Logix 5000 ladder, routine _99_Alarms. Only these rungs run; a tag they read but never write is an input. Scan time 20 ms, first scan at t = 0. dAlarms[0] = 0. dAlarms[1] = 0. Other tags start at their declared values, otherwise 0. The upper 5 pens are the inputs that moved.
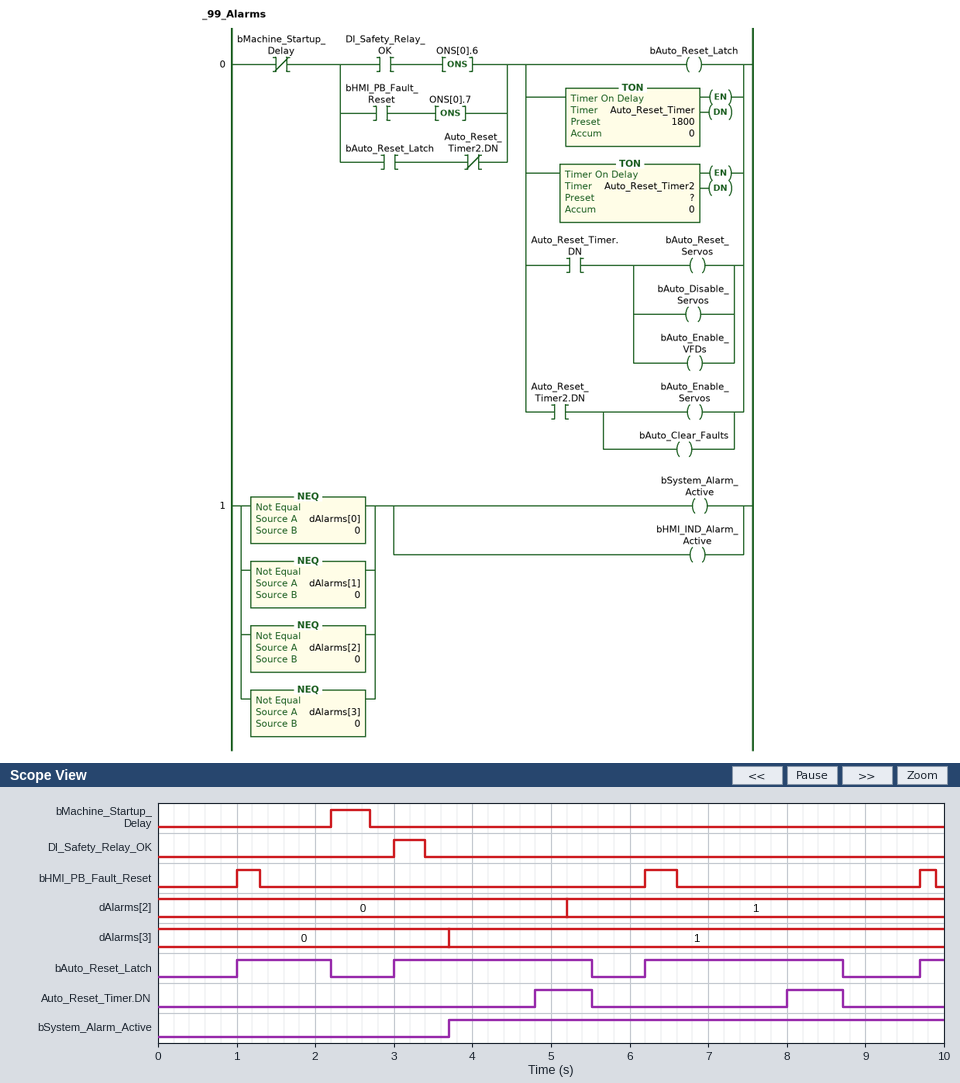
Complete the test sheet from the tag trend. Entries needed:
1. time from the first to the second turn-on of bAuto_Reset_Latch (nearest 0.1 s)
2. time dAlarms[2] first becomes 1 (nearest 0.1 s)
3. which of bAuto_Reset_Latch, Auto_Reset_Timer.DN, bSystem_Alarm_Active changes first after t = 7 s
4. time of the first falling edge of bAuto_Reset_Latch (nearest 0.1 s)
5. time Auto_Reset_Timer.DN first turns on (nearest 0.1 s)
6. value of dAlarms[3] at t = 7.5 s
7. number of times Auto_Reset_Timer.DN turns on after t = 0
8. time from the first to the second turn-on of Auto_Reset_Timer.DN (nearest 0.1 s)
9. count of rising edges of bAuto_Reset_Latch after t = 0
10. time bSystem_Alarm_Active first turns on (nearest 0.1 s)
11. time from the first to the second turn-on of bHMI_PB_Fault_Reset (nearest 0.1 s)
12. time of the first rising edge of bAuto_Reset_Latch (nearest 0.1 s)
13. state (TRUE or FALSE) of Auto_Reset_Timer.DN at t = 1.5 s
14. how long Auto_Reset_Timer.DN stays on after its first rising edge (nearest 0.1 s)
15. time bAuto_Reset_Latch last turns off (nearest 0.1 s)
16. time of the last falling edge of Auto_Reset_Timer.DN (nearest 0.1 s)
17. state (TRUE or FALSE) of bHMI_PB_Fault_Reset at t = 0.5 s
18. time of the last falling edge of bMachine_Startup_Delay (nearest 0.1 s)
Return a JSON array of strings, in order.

["2.0 s", "5.2 s", "Auto_Reset_Timer.DN", "2.2 s", "4.8 s", "1", "2", "3.2 s", "4", "3.7 s", "5.2 s", "1.0 s", "FALSE", "0.7 s", "8.7 s", "8.7 s", "FALSE", "2.7 s"]
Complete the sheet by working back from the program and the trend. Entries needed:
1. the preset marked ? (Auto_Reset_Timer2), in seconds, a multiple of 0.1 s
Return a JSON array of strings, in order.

["2.5 s"]
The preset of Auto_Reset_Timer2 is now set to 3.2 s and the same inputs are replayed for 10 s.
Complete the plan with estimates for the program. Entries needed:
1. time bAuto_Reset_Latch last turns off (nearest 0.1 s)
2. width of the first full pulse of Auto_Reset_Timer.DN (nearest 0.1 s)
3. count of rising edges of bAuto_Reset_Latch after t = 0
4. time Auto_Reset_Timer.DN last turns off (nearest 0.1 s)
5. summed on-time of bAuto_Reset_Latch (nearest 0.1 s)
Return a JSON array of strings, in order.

["6.2 s", "1.4 s", "3", "6.2 s", "4.7 s"]
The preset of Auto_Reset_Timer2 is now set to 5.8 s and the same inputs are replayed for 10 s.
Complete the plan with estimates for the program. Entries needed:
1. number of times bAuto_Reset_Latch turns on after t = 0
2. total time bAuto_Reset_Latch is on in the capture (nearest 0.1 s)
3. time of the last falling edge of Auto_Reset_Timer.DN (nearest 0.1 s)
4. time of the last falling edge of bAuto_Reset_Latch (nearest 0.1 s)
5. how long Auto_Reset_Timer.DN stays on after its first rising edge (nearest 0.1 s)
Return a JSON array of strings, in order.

["3", "7.3 s", "8.8 s", "8.8 s", "4.0 s"]
